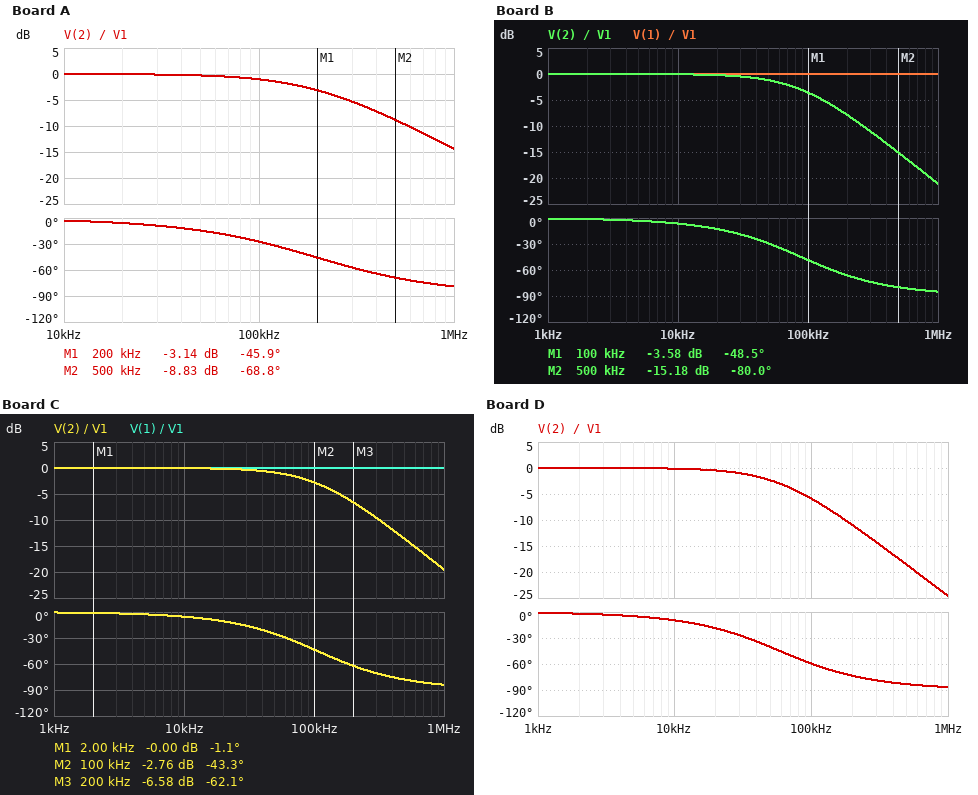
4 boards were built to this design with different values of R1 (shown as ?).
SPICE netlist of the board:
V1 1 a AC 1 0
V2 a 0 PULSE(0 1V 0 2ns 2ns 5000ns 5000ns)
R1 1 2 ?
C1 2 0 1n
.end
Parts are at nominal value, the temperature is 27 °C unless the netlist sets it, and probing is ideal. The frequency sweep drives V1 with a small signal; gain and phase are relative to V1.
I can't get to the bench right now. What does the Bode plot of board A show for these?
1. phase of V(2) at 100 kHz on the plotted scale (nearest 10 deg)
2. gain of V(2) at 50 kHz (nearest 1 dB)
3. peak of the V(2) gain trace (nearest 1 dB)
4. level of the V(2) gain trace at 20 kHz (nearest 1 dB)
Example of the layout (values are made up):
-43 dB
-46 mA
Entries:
-30 deg
0 dB
0 dB
0 dB
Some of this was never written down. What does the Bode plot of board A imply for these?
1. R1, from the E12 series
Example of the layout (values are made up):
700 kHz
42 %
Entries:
820 Ω
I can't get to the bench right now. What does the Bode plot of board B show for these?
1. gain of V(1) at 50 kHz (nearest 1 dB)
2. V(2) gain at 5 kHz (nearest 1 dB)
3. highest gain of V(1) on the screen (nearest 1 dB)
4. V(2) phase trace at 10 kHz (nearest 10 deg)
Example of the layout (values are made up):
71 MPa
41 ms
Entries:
0 dB
0 dB
0 dB
-10 deg
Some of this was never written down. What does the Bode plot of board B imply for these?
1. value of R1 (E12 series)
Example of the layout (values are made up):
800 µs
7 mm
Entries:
1.8 kΩ
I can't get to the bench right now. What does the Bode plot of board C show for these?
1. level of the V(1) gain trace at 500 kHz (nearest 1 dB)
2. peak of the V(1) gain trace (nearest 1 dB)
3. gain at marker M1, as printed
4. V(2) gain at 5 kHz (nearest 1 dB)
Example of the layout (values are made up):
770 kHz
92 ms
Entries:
0 dB
0 dB
-0.00 dB
0 dB
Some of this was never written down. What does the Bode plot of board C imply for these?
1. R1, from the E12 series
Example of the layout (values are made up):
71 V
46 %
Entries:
1.5 kΩ
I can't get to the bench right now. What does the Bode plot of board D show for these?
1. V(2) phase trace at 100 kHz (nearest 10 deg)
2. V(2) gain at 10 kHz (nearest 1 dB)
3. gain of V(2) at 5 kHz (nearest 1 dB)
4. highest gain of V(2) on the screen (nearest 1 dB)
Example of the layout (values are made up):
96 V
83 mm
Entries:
-60 deg
0 dB
0 dB
0 dB
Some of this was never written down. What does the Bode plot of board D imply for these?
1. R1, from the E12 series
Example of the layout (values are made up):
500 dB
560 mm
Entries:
2.7 kΩ
